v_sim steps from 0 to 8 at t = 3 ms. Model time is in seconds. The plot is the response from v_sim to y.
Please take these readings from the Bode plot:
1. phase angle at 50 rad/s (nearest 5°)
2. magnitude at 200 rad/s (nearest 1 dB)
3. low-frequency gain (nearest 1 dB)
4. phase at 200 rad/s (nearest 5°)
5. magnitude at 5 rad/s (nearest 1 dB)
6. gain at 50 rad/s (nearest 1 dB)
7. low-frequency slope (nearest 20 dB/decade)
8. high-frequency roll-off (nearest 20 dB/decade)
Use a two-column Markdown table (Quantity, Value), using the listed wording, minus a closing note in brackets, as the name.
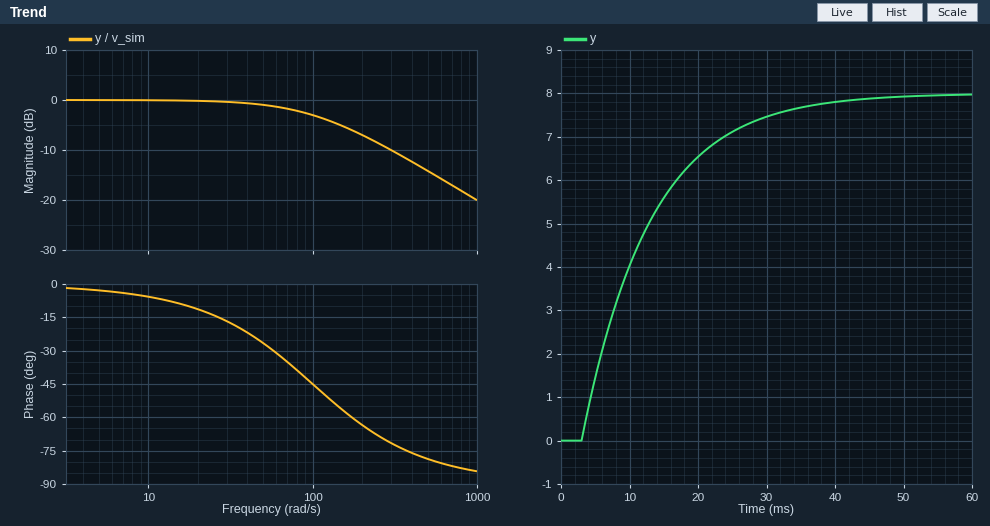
| Quantity | Value |
|---|---|
| phase angle at 50 rad/s | -25° |
| magnitude at 200 rad/s | -7 dB |
| low-frequency gain | 0 dB |
| phase at 200 rad/s | -65° |
| magnitude at 5 rad/s | 0 dB |
| gain at 50 rad/s | -1 dB |
| low-frequency slope | 0 dB/decade |
| high-frequency roll-off | -20 dB/decade |
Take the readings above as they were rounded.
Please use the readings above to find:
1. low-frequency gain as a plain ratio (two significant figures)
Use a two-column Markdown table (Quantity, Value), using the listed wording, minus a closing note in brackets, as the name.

| Quantity | Value |
|---|---|
| low-frequency gain as a plain ratio | 1.0 |
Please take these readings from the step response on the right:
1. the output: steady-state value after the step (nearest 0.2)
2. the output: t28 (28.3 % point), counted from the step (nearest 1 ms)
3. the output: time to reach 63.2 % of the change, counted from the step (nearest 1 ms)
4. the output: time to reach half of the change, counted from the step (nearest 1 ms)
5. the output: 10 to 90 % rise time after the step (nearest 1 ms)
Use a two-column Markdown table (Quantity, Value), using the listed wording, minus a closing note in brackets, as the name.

| Quantity | Value |
|---|---|
| the output: steady-state value after the step | 8.0 |
| the output: t28 (28.3 % point), counted from the step | 3 ms |
| the output: time to reach 63.2 % of the change, counted from the step | 10 ms |
| the output: time to reach half of the change, counted from the step | 7 ms |
| the output: 10 to 90 % rise time after the step | 22 ms |
